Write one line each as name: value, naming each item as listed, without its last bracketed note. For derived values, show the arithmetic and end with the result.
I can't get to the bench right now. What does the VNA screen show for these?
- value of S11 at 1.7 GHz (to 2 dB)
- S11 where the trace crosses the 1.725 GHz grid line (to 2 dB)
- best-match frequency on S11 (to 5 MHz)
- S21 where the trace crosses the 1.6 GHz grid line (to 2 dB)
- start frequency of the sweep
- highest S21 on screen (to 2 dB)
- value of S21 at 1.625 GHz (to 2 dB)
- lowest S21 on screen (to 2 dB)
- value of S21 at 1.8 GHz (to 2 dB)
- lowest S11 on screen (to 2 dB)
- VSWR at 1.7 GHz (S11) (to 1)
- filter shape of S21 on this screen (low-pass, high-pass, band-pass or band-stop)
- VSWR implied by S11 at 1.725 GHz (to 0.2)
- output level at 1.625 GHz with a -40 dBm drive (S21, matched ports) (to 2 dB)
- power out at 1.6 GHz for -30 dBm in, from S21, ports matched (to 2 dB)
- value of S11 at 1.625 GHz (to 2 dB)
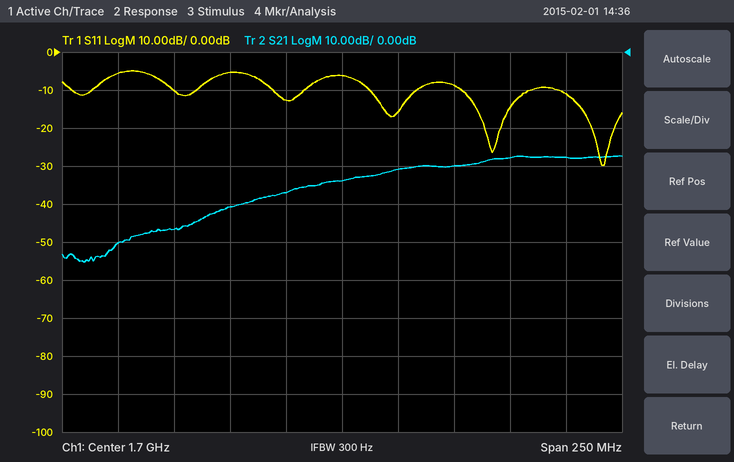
value of S11 at 1.7 GHz: -6 dB
S11 where the trace crosses the 1.725 GHz grid line: -16 dB
best-match frequency on S11: 1.815 GHz
S21 where the trace crosses the 1.6 GHz grid line: -50 dB
start frequency of the sweep: 1.575 GHz
highest S21 on screen: -28 dB
value of S21 at 1.625 GHz: -46 dB
lowest S21 on screen: -56 dB
value of S21 at 1.8 GHz: -28 dB
lowest S11 on screen: -30 dB
VSWR at 1.7 GHz (S11): |Γ| = 10^(-6/20) = 0.5012; VSWR = (1 + 0.5012)/(1 − 0.5012) ≈ 3
filter shape of S21 on this screen: high-pass
VSWR implied by S11 at 1.725 GHz: |Γ| = 10^(-16/20) = 0.1585; VSWR = (1 + 0.1585)/(1 − 0.1585) ≈ 1.4
output level at 1.625 GHz with a -40 dBm drive (S21, matched ports): -40 dBm + (-46 dB) = -86 dBm
power out at 1.6 GHz for -30 dBm in, from S21, ports matched: -30 dBm + (-50 dB) = -80 dBm
value of S11 at 1.625 GHz: -10 dB
